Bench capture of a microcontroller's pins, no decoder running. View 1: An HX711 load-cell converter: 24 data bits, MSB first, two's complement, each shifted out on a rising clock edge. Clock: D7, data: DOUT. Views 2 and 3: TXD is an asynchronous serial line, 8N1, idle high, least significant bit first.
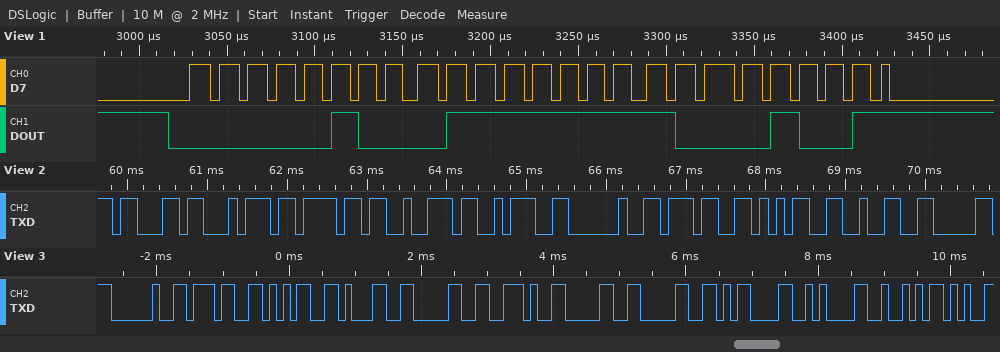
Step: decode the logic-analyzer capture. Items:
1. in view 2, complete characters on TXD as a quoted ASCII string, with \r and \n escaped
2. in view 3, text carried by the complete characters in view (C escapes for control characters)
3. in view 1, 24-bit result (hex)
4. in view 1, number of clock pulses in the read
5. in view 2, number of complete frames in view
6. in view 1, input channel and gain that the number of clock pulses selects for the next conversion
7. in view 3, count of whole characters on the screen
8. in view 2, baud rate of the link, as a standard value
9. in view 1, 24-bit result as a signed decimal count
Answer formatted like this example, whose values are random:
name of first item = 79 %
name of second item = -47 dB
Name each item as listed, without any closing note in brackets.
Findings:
in view 2, complete characters on TXD as a quoted ASCII string, with \r and \n escaped = "ctor: 752"
in view 3, text carried by the complete characters in view = " 7510.00\r\nR"
in view 1, 24-bit result = 0x047F89
in view 1, number of clock pulses in the read = 25
in view 2, number of complete frames in view = 9
in view 1, input channel and gain that the number of clock pulses selects for the next conversion = channel A, gain 128
in view 3, count of whole characters on the screen = 11
in view 2, baud rate of the link, as a standard value = 9600 baud
in view 1, 24-bit result as a signed decimal count = 294793
